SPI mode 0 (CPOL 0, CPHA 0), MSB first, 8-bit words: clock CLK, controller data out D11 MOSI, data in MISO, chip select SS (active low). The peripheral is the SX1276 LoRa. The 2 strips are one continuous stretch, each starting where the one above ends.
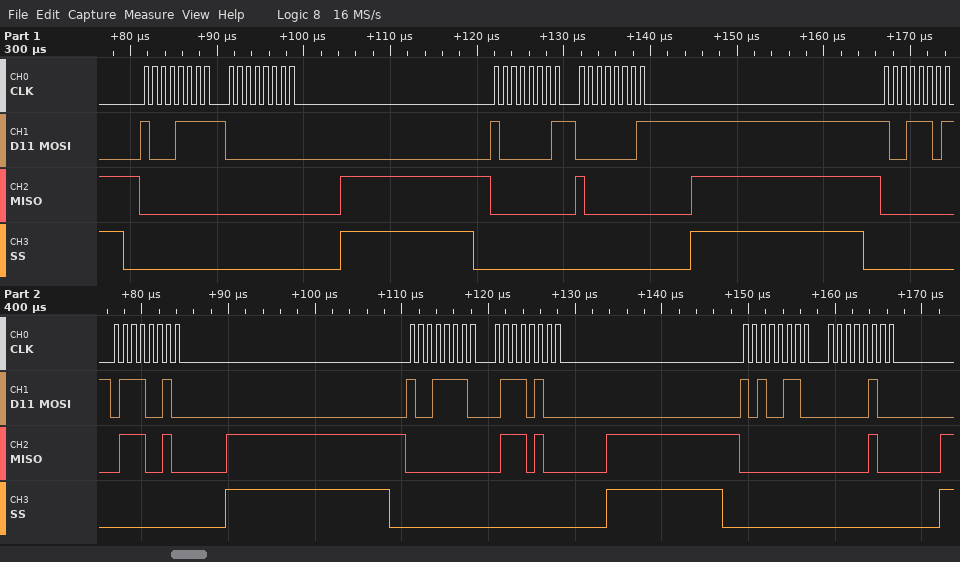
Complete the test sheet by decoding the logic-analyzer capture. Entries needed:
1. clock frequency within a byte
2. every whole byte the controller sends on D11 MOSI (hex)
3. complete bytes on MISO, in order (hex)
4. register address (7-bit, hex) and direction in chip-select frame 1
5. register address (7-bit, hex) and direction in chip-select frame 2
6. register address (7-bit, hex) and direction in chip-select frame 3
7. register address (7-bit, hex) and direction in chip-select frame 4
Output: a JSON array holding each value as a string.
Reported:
["1 MHz", "8F 00 81 01 9D 72 9E 74 A6 04", "00 00 00 80 00 72 00 74 00 04", "0x0F write", "0x01 write", "0x1D write", "0x1E write"]
